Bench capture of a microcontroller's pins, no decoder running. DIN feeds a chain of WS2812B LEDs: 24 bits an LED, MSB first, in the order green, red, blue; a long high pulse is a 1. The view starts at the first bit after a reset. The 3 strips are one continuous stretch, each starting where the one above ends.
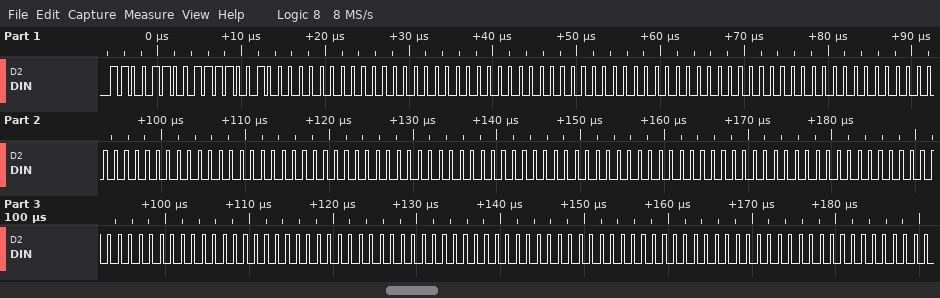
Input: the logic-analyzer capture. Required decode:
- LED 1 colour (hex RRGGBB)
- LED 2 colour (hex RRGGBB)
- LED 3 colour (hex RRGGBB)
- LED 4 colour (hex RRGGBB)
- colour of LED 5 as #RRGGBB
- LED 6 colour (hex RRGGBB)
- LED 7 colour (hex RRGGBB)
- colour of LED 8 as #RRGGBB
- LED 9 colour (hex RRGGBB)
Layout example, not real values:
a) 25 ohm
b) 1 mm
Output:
a) #F2CC00
b) #000000
c) #000000
d) #000000
e) #000000
f) #000000
g) #000000
h) #000000
i) #000000
